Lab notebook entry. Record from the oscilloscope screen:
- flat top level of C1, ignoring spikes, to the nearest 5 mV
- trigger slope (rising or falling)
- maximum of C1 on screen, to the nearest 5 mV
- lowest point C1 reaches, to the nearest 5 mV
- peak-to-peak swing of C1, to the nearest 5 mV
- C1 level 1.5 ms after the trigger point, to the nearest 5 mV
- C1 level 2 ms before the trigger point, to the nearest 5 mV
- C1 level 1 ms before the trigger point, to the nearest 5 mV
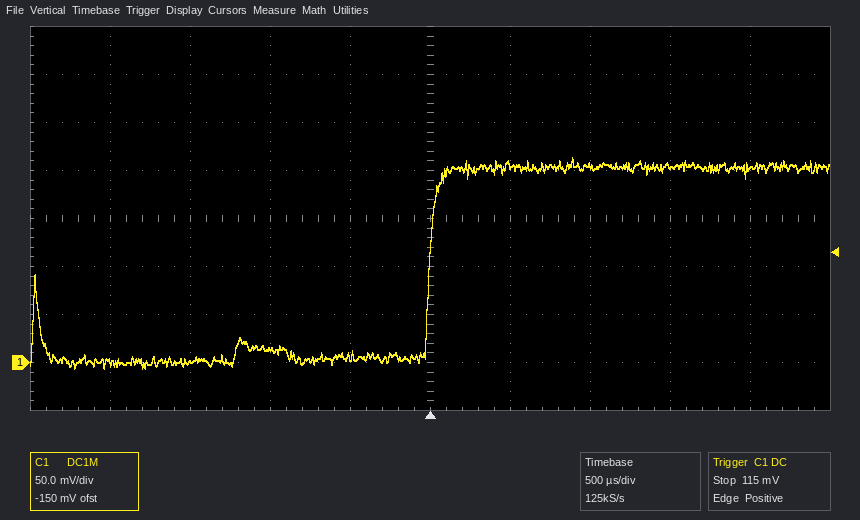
205 mV
rising
215 mV
-5 mV
220 mV
205 mV
0 mV
15 mV
